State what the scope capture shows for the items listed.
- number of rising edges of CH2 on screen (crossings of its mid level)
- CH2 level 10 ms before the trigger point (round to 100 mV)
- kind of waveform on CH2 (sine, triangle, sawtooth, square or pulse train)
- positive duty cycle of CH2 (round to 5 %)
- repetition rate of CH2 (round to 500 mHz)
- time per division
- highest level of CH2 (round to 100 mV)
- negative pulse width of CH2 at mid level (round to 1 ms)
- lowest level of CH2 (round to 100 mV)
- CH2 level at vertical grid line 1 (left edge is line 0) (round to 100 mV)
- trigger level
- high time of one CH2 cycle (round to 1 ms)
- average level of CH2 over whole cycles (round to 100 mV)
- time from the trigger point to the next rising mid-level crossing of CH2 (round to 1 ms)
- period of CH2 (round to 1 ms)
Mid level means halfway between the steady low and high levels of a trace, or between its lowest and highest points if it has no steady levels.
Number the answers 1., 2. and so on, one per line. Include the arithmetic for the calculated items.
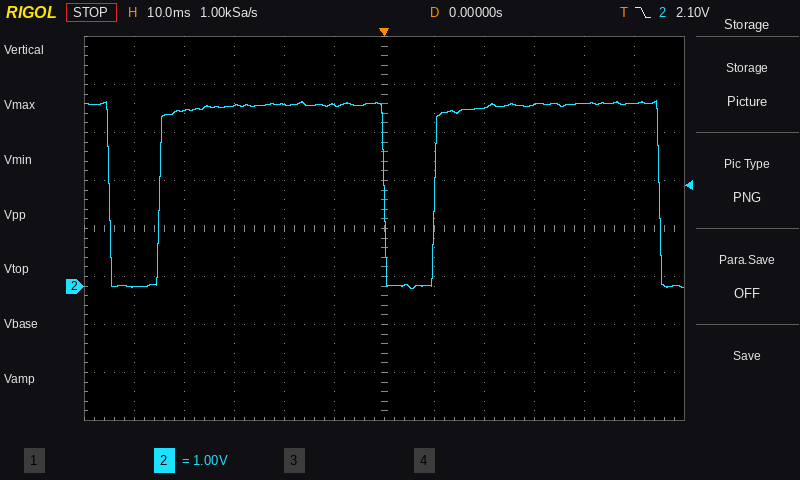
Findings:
1. 2
2. 3.8 V
3. pulse train
4. 45 ms / 55 ms ≈ 81.8 %, so 80 % to the nearest 5 %
5. 1 / 55 ms ≈ 18.2 Hz, so 18.0 Hz to the nearest 500 mHz
6. 10 ms
7. 3.9 V
8. 10 ms
9. -100 mV
10. 0.0 V
11. 2.10 V
12. 45 ms
13. -100 mV + 0.8 × (3.9 V − (-100 mV)) ≈ 3.1 V
14. 10 ms
15. 55 ms
